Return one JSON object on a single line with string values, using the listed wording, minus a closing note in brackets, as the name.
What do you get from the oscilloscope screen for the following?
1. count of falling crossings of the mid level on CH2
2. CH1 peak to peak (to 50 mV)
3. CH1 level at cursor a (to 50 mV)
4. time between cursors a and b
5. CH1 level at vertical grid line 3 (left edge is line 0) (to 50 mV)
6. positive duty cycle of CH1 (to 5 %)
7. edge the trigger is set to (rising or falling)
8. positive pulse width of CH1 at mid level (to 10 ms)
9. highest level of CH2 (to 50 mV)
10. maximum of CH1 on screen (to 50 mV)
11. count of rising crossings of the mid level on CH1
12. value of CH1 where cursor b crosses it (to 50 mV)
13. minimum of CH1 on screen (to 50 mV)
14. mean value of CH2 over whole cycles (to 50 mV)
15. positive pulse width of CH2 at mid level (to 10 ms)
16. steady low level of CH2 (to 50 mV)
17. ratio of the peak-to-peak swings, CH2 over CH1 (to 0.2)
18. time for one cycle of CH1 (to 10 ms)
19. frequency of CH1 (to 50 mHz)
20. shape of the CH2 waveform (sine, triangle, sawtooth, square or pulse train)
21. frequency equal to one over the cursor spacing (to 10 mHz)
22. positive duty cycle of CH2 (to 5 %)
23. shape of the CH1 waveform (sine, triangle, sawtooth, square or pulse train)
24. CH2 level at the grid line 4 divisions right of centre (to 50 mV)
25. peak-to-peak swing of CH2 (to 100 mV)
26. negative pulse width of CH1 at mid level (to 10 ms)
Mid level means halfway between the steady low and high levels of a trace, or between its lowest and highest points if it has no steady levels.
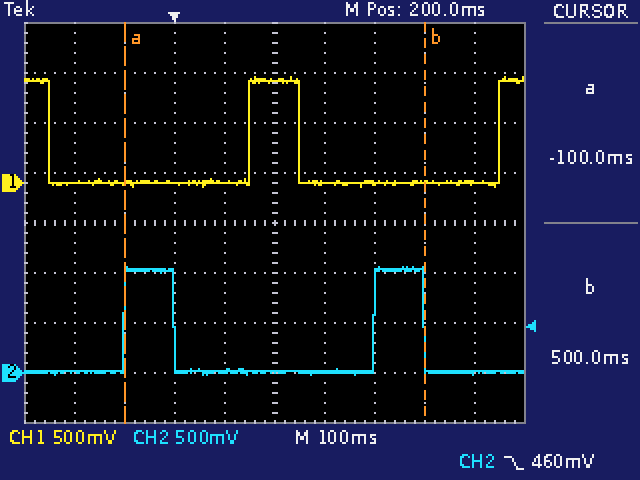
{"count of falling crossings of the mid level on CH2": "2", "CH1 peak to peak": "1.10 V", "CH1 level at cursor a": "0 mV", "time between cursors a and b": "600 ms", "CH1 level at vertical grid line 3 (left edge is line 0)": "0 mV", "positive duty cycle of CH1": "20 %", "edge the trigger is set to": "falling", "positive pulse width of CH1 at mid level": "100 ms", "highest level of CH2": "1.05 V", "maximum of CH1 on screen": "1.05 V", "count of rising crossings of the mid level on CH1": "2", "value of CH1 where cursor b crosses it": "0 mV", "minimum of CH1 on screen": "-50 mV", "mean value of CH2 over whole cycles": "200 mV", "positive pulse width of CH2 at mid level": "100 ms", "steady low level of CH2": "0 mV", "ratio of the peak-to-peak swings, CH2 over CH1": "1.0", "time for one cycle of CH1": "500 ms", "frequency of CH1": "2.00 Hz", "shape of the CH2 waveform": "pulse train", "frequency equal to one over the cursor spacing": "1.67 Hz", "positive duty cycle of CH2": "20 %", "shape of the CH1 waveform": "pulse train", "CH2 level at the grid line 4 divisions right of centre": "0 mV", "peak-to-peak swing of CH2": "1.10 V", "negative pulse width of CH1 at mid level": "400 ms"}
